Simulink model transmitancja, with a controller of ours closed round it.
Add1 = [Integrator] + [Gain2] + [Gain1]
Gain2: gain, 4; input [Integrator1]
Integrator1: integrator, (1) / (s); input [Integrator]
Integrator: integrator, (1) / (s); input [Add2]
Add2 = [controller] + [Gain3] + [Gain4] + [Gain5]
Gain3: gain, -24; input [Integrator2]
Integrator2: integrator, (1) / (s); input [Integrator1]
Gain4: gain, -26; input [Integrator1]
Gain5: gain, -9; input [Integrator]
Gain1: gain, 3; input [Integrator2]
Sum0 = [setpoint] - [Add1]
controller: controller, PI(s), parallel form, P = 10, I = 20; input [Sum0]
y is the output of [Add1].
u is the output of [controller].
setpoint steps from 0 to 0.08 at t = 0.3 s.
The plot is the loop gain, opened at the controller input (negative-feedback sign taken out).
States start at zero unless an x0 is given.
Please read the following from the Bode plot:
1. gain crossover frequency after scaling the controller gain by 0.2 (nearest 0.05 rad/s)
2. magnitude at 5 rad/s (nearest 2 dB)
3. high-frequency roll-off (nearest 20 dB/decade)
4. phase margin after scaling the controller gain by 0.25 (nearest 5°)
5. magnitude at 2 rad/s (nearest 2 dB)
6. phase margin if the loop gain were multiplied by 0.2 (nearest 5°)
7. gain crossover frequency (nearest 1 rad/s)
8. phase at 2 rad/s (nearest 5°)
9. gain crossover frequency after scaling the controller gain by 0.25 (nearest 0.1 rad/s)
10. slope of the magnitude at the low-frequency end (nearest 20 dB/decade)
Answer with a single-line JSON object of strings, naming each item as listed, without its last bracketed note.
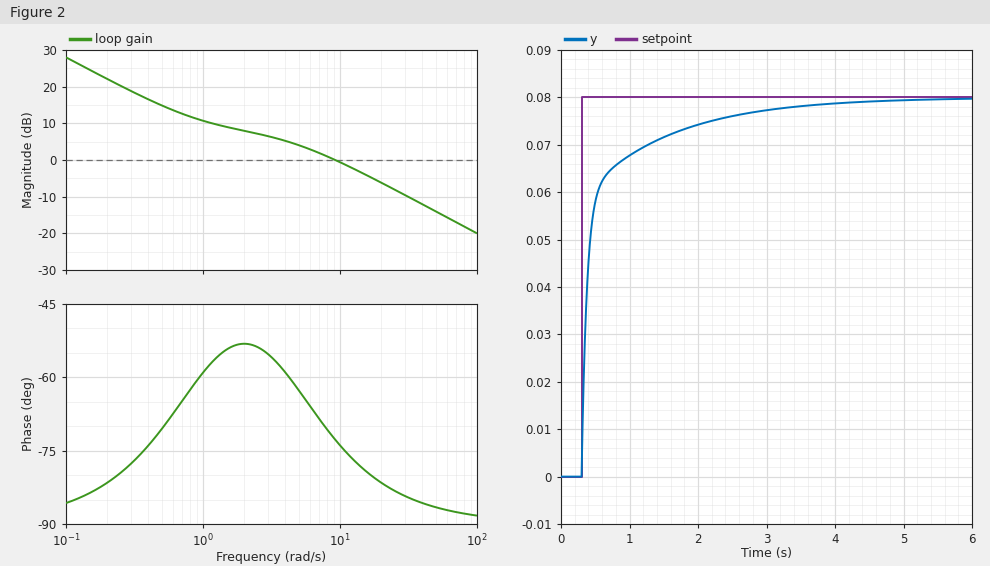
{"gain crossover frequency after scaling the controller gain by 0.2": "0.55 rad/s", "magnitude at 5 rad/s": "4 dB", "high-frequency roll-off": "-20 dB/decade", "phase margin after scaling the controller gain by 0.25": "115°", "magnitude at 2 rad/s": "8 dB", "phase margin if the loop gain were multiplied by 0.2": "110°", "gain crossover frequency": "9 rad/s", "phase at 2 rad/s": "-55°", "gain crossover frequency after scaling the controller gain by 0.25": "0.8 rad/s", "slope of the magnitude at the low-frequency end": "-20 dB/decade"}
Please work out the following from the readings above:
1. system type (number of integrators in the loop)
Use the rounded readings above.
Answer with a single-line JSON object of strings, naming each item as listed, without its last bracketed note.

{"system type": "1"}
